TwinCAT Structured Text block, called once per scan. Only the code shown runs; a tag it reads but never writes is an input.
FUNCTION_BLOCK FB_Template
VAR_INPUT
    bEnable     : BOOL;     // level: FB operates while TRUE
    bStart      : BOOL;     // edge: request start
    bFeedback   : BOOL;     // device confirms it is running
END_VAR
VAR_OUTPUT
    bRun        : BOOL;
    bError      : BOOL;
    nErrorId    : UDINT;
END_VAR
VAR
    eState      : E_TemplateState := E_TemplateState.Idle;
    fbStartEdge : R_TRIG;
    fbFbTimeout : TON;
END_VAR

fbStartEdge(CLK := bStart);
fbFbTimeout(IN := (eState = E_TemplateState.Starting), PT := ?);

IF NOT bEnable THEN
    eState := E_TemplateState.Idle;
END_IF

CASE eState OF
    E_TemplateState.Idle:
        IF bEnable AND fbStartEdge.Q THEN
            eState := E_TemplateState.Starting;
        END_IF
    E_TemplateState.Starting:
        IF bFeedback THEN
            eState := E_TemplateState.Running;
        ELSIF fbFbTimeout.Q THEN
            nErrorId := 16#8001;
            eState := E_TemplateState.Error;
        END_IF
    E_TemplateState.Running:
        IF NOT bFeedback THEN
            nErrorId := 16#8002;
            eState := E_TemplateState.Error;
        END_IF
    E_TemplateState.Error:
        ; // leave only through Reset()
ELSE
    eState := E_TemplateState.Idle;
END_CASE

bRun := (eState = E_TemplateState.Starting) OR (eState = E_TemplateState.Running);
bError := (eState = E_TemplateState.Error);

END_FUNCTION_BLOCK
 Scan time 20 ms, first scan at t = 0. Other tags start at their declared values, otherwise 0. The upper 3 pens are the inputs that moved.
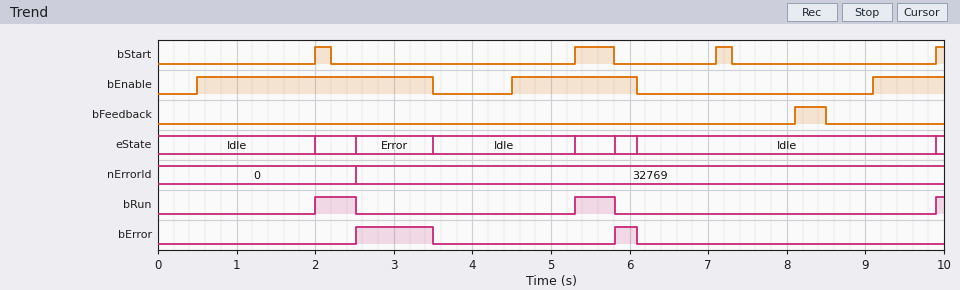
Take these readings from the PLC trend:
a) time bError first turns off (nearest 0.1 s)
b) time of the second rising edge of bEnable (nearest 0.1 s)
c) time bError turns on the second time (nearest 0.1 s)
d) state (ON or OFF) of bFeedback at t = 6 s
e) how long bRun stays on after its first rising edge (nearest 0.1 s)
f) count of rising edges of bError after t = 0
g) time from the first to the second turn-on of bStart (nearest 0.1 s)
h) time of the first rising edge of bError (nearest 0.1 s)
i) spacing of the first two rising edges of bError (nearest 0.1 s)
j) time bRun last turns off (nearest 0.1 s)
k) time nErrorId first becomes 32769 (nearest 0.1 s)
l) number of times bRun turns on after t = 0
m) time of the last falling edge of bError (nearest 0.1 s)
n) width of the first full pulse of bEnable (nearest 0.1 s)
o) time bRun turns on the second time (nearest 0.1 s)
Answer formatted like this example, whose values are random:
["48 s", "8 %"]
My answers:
["3.5 s", "4.5 s", "5.8 s", "OFF", "0.5 s", "2", "3.3 s", "2.5 s", "3.3 s", "5.8 s", "2.5 s", "3", "6.1 s", "3.0 s", "5.3 s"]
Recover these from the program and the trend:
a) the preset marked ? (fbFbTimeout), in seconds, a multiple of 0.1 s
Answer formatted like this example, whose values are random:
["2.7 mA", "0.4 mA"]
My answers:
["0.5 s"]
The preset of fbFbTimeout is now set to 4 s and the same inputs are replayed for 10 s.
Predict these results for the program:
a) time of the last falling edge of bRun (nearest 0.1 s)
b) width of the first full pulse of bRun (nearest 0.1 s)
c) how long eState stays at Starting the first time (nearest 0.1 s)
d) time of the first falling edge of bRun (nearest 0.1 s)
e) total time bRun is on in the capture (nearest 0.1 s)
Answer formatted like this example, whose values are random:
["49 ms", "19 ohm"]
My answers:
["6.1 s", "1.5 s", "1.5 s", "3.5 s", "2.4 s"]
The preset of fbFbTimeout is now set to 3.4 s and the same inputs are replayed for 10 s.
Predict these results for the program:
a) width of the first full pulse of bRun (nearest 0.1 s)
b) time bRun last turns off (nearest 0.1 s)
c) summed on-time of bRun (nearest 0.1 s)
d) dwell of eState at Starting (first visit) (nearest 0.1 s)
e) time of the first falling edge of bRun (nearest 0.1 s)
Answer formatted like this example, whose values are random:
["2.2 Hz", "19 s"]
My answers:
["1.5 s", "6.1 s", "2.4 s", "1.5 s", "3.5 s"]
